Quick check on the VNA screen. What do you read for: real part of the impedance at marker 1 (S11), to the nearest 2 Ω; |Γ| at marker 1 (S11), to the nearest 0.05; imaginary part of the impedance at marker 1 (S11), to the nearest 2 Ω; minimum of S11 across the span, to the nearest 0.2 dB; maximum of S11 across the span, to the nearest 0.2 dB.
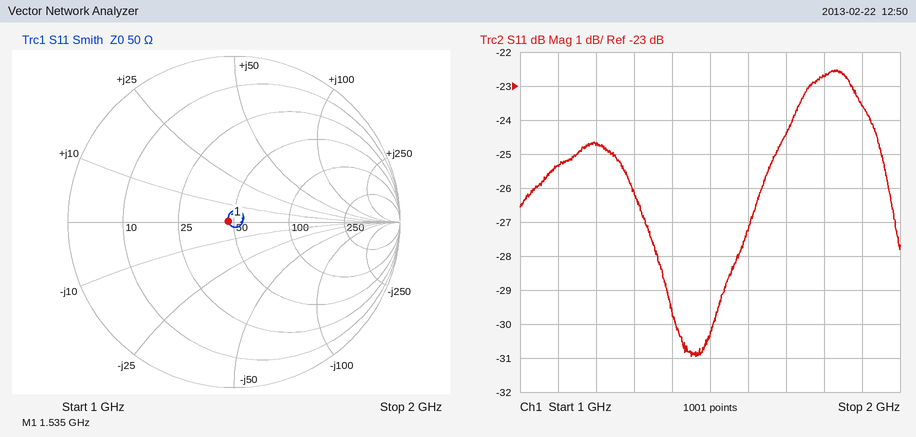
46 Ω
0.05
0 Ω
-31.0 dB
-22.6 dB
